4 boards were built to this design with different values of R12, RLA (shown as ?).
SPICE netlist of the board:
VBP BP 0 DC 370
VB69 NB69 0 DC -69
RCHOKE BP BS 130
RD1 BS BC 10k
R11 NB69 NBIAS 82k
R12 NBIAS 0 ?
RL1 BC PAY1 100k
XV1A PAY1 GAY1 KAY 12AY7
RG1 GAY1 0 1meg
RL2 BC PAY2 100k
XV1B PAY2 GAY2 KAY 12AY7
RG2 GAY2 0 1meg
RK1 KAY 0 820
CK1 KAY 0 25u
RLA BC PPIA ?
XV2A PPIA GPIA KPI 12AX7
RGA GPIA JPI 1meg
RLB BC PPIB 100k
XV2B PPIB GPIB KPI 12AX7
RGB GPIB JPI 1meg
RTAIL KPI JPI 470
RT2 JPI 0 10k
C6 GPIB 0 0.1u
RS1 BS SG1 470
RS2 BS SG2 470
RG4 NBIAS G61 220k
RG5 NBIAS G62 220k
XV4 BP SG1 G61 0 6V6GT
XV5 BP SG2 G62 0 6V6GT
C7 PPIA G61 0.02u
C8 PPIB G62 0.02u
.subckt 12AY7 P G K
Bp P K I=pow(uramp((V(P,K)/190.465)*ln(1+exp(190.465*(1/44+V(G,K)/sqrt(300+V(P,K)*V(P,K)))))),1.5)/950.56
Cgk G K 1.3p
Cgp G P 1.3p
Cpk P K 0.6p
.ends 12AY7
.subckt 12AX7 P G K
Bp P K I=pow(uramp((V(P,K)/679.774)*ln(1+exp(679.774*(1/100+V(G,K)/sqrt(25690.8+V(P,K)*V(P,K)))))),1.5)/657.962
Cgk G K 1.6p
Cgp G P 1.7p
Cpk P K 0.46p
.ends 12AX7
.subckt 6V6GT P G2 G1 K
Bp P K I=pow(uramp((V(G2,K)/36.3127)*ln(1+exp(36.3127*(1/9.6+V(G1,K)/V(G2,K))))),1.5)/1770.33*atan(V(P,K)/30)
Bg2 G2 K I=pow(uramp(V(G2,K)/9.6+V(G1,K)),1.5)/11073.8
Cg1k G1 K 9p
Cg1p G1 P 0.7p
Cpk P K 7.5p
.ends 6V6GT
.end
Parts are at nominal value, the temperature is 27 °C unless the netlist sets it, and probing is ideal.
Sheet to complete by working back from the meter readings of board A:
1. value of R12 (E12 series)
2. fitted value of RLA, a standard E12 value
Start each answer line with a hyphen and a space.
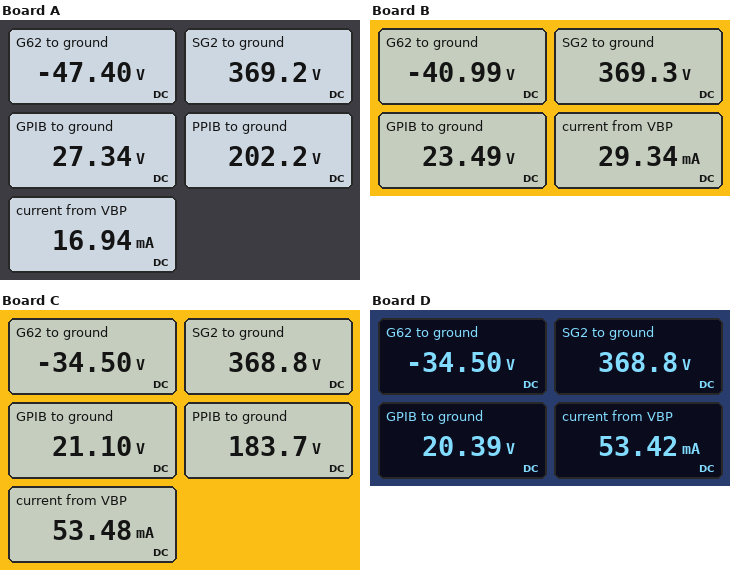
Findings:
- 180 kΩ
- 47 kΩ
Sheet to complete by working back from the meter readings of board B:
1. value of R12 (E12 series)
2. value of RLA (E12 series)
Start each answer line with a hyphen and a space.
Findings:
- 120 kΩ
- 120 kΩ
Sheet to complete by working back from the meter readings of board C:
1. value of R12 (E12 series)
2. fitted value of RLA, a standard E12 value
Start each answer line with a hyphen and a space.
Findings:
- 82 kΩ
- 220 kΩ
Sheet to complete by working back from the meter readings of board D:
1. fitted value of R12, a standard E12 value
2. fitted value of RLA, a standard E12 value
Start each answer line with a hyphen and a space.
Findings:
- 82 kΩ
- 270 kΩ
